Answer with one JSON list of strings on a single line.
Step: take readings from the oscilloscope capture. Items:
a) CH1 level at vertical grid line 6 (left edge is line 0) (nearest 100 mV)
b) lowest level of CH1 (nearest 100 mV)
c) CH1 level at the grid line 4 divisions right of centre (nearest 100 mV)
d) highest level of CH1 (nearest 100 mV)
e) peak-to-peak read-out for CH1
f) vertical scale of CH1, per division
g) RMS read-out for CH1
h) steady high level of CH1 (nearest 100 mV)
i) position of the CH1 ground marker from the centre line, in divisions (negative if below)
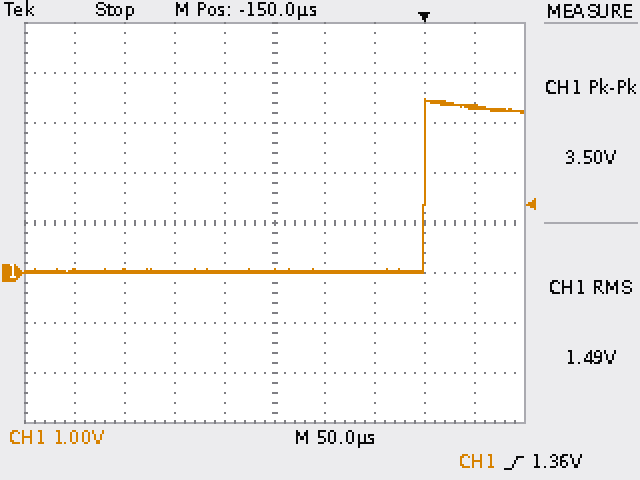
["0.0 V", "0.0 V", "3.3 V", "3.5 V", "3.50 V", "1 V", "1.49 V", "3.3 V", "-1.0 div"]
